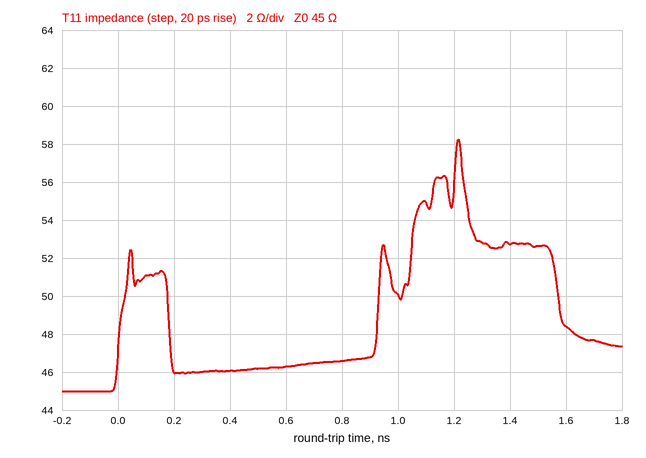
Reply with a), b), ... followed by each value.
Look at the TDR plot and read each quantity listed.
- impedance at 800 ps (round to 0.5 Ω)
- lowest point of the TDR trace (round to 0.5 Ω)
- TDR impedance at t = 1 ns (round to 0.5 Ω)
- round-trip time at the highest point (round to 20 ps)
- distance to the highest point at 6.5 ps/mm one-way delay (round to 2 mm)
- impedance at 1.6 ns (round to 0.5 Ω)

a) 46.5 Ω
b) 45.0 Ω
c) 50.0 Ω
d) 1.22 ns
e) 94 mm
f) 48.5 Ω
